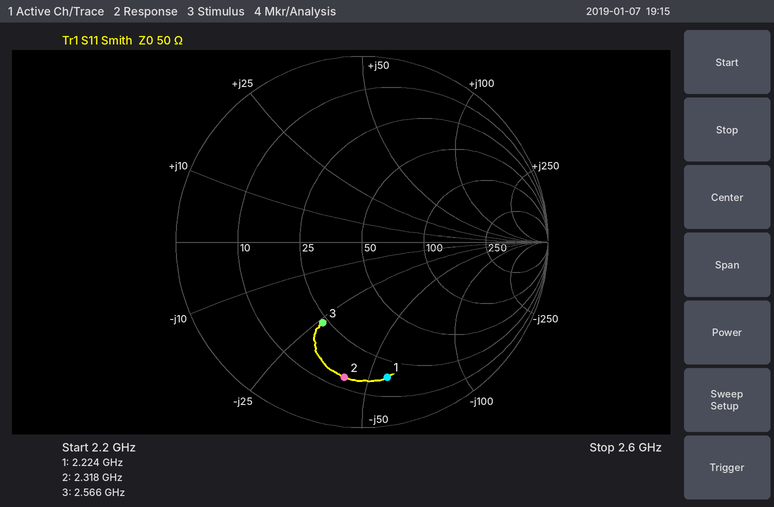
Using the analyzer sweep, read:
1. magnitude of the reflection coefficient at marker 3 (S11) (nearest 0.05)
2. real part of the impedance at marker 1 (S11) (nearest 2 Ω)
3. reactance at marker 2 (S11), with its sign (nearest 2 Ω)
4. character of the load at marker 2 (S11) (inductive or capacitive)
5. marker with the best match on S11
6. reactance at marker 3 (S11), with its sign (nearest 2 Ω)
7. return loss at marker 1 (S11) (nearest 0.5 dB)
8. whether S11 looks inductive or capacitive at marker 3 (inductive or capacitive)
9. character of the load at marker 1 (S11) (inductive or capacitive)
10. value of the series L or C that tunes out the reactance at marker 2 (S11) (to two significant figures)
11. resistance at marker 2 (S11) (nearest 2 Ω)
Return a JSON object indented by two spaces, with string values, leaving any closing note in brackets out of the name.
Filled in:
{
  "magnitude of the reflection coefficient at marker 3 (S11)": "0.50",
  "real part of the impedance at marker 1 (S11)": "18 Ω",
  "reactance at marker 2 (S11), with its sign": "-42 Ω",
  "character of the load at marker 2 (S11)": "capacitive",
  "marker with the best match on S11": "marker 3",
  "reactance at marker 3 (S11), with its sign": "-26 Ω",
  "return loss at marker 1 (S11)": "2.5 dB",
  "whether S11 looks inductive or capacitive at marker 3": "capacitive",
  "character of the load at marker 1 (S11)": "capacitive",
  "value of the series L or C that tunes out the reactance at marker 2 (S11)": "2.9 nH",
  "resistance at marker 2 (S11)": "14 Ω"
}
